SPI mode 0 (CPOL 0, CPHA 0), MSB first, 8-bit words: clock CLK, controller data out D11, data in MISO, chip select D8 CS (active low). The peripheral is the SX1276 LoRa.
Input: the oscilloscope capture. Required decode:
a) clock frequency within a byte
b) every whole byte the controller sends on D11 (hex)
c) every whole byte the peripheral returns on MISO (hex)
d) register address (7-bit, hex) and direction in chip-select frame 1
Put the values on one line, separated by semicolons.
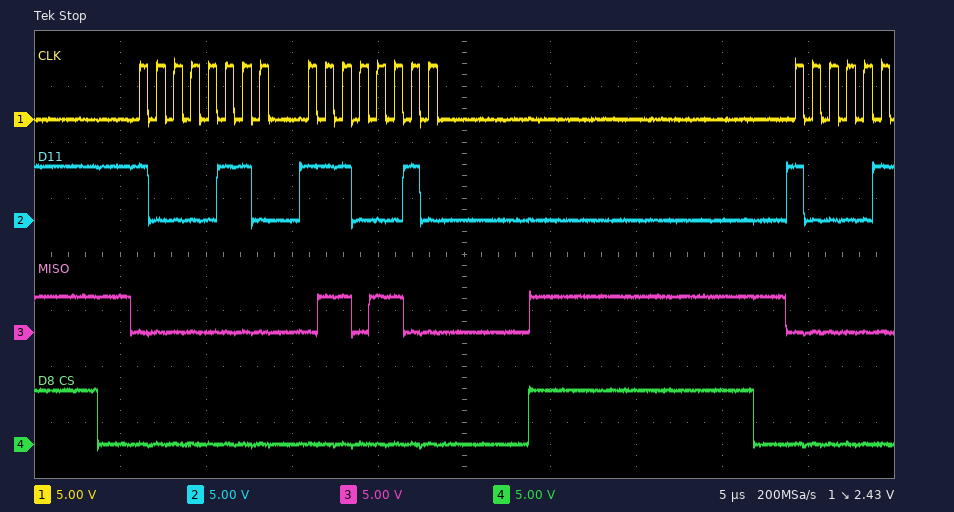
1 MHz; 86 E2; 00 6C; 0x06 write
